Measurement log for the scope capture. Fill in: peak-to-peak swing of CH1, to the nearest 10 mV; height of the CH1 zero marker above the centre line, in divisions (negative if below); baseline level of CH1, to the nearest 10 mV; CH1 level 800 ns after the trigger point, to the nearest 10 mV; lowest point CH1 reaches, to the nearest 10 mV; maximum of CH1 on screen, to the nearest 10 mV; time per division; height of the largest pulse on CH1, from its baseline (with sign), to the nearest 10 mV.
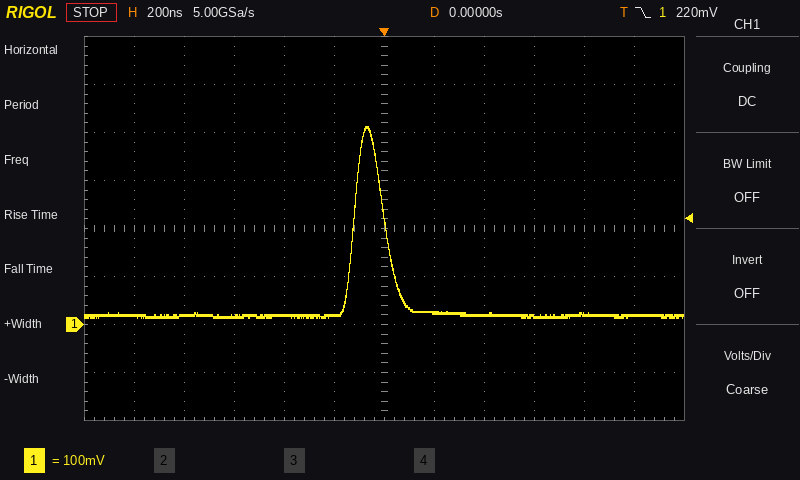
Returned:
400 mV
-2.0 div
20 mV
20 mV
10 mV
410 mV
200 ns
+390 mV
